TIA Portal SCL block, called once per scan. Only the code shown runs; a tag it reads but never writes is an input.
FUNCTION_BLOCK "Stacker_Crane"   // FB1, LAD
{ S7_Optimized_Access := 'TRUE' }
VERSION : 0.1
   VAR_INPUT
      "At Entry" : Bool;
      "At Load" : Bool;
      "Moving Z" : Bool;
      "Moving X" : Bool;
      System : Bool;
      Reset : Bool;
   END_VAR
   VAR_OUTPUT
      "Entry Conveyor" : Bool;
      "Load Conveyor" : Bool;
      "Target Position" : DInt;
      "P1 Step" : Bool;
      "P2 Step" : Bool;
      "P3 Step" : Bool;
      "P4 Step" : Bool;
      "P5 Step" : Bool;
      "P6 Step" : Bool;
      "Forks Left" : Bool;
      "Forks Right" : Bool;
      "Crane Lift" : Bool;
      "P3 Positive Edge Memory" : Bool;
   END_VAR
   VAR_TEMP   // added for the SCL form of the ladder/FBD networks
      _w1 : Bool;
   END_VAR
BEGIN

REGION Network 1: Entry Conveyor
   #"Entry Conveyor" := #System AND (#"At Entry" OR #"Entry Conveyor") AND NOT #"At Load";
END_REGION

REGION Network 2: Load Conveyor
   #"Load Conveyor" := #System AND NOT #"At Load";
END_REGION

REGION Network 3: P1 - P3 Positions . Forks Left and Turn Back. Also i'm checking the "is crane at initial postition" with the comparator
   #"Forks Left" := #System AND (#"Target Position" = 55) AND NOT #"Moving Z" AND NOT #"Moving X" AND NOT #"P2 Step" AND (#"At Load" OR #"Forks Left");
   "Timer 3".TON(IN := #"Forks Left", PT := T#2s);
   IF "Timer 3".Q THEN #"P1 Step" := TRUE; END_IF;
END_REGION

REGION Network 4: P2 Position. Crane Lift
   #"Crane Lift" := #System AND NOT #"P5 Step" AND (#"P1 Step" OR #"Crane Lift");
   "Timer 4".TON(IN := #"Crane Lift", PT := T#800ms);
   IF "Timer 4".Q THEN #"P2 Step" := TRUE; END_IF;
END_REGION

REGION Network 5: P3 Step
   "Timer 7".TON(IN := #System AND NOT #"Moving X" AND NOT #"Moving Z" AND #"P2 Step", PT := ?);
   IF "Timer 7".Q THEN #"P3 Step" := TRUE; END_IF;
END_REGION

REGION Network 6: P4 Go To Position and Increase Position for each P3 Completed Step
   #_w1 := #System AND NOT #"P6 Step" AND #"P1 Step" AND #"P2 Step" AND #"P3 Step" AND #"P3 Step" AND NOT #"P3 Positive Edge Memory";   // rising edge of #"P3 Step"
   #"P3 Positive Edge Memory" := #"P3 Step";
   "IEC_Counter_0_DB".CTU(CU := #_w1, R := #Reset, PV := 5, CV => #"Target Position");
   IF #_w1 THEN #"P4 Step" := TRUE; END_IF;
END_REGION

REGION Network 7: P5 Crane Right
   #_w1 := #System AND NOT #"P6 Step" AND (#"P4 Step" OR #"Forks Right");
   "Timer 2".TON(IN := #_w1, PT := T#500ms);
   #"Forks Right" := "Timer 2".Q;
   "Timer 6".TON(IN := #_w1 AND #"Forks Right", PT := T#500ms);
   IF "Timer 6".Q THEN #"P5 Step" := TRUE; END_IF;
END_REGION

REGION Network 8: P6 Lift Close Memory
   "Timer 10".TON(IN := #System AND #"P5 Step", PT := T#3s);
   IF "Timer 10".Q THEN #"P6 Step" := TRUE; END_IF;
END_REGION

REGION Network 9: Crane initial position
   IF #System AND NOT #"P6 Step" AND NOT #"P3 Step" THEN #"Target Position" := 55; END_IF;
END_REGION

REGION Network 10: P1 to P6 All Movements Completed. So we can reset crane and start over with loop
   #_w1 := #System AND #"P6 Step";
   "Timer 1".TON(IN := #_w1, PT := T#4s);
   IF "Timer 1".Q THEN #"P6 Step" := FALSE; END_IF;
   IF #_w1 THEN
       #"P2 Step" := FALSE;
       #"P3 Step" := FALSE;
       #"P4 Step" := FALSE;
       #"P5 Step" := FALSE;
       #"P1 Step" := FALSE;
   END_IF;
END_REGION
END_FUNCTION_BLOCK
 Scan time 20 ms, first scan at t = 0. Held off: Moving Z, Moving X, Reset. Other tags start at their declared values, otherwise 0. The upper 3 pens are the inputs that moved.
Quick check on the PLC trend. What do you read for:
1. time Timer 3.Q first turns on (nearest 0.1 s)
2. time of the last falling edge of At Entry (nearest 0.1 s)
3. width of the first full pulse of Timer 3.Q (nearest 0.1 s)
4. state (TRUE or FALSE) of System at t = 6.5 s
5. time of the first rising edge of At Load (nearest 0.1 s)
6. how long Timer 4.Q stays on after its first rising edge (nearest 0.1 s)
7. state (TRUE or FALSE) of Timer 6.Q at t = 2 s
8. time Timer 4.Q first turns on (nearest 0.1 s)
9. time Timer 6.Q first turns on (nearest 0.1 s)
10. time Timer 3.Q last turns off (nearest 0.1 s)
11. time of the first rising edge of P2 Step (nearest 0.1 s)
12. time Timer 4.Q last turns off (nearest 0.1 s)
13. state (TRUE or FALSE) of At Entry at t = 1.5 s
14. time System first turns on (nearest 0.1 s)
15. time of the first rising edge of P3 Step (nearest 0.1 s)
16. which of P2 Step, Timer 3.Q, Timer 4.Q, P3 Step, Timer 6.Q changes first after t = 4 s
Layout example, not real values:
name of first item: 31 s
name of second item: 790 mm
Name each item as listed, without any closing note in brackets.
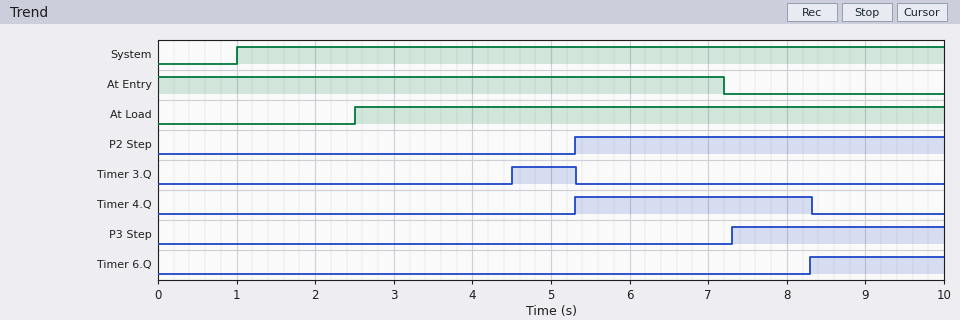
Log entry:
time Timer 3.Q first turns on: 4.5 s
time of the last falling edge of At Entry: 7.2 s
width of the first full pulse of Timer 3.Q: 0.8 s
state (TRUE or FALSE) of System at t = 6.5 s: TRUE
time of the first rising edge of At Load: 2.5 s
how long Timer 4.Q stays on after its first rising edge: 3.0 s
state (TRUE or FALSE) of Timer 6.Q at t = 2 s: FALSE
time Timer 4.Q first turns on: 5.3 s
time Timer 6.Q first turns on: 8.3 s
time Timer 3.Q last turns off: 5.3 s
time of the first rising edge of P2 Step: 5.3 s
time Timer 4.Q last turns off: 8.3 s
state (TRUE or FALSE) of At Entry at t = 1.5 s: TRUE
time System first turns on: 1.0 s
time of the first rising edge of P3 Step: 7.3 s
which of P2 Step, Timer 3.Q, Timer 4.Q, P3 Step, Timer 6.Q changes first after t = 4 s: Timer 3.Q
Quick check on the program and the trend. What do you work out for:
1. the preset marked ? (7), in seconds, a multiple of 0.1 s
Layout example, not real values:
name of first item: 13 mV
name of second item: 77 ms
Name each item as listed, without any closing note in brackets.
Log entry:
the preset marked ? (7), in seconds, a multiple of 0.1 s: 2.0 s
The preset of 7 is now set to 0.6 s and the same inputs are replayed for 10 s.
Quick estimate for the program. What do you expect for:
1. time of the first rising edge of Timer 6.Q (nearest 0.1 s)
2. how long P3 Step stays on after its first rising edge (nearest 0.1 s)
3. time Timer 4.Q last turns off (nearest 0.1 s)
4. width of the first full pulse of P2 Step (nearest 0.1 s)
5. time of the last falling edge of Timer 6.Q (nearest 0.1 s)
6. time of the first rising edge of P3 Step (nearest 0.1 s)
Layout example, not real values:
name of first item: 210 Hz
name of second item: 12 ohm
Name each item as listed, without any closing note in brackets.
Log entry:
time of the first rising edge of Timer 6.Q: 6.9 s
how long P3 Step stays on after its first rising edge: 4.0 s
time Timer 4.Q last turns off: 6.9 s
width of the first full pulse of P2 Step: 4.6 s
time of the last falling edge of Timer 6.Q: 9.9 s
time of the first rising edge of P3 Step: 5.9 s
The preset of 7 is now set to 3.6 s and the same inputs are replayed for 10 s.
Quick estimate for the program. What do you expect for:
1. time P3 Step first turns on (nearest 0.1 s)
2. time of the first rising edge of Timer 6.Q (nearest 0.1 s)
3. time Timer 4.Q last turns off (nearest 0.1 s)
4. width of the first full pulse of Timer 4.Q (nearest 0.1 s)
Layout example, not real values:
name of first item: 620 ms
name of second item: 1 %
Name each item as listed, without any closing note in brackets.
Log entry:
time P3 Step first turns on: 8.9 s
time of the first rising edge of Timer 6.Q: 9.9 s
time Timer 4.Q last turns off: 9.9 s
width of the first full pulse of Timer 4.Q: 4.6 s
